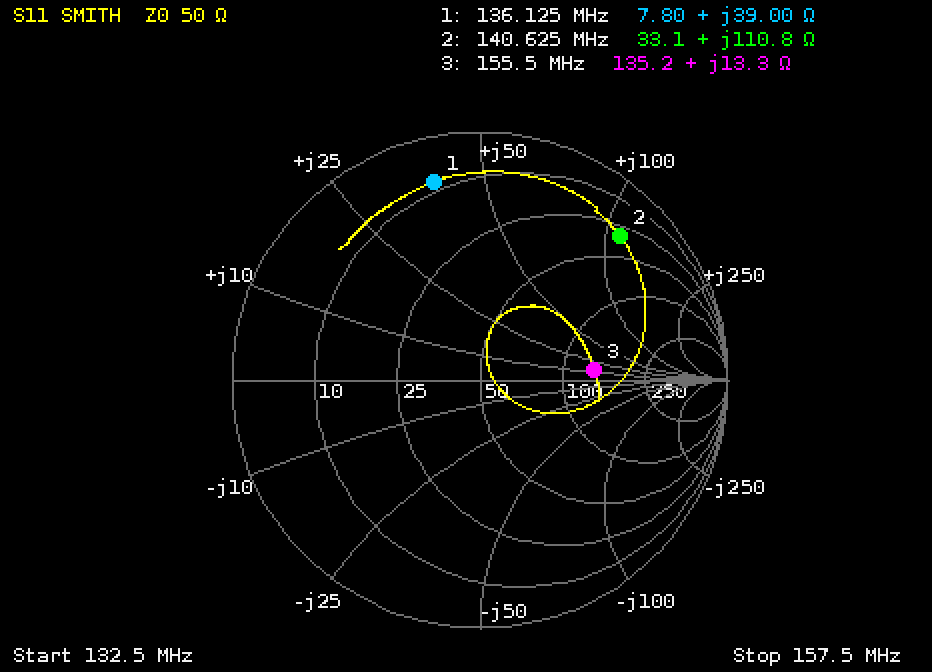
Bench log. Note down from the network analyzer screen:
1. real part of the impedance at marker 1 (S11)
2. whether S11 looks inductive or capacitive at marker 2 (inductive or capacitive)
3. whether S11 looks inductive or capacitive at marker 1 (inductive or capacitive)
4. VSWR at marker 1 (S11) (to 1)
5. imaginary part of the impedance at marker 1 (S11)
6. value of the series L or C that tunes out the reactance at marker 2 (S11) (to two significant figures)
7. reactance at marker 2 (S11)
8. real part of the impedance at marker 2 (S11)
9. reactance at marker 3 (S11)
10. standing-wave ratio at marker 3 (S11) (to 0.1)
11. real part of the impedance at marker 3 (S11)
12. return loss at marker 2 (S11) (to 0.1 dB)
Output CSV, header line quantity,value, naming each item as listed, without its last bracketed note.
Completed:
quantity,value
real part of the impedance at marker 1,7.80 Ω
whether S11 looks inductive or capacitive at marker 2,inductive
whether S11 looks inductive or capacitive at marker 1,inductive
VSWR at marker 1 (S11),10
imaginary part of the impedance at marker 1,+39.00 Ω
value of the series L or C that tunes out the reactance at marker 2 (S11),10 pF
reactance at marker 2,+110.8 Ω
real part of the impedance at marker 2,33.1 Ω
reactance at marker 3,+13.3 Ω
standing-wave ratio at marker 3 (S11),2.7
real part of the impedance at marker 3,135.2 Ω
return loss at marker 2 (S11),1.8 dB
